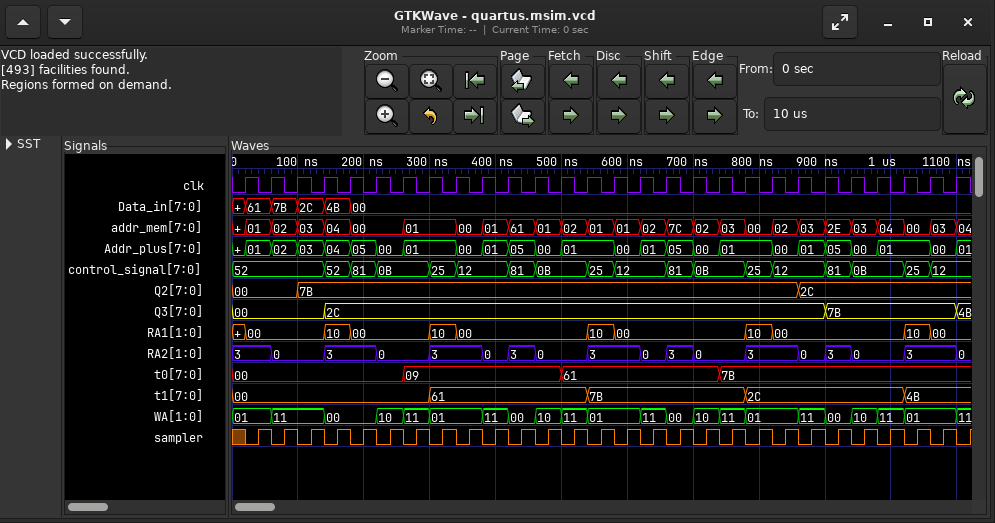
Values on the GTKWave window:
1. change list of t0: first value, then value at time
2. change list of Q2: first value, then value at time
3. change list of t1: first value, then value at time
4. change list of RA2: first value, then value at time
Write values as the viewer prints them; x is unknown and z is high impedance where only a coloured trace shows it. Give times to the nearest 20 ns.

00, 09 at 260 ns, 61 at 500 ns, 7B at 740 ns
00, 7B at 100 ns, 2C at 860 ns
00, 61 at 300 ns, 7B at 540 ns, 2C at 780 ns, 4B at 1020 ns
3, 0 at 60 ns, 3 at 140 ns, 0 at 220 ns, 3 at 300 ns, 0 at 380 ns, 3 at 420 ns, 0 at 460 ns, 3 at 540 ns, 0 at 620 ns, 3 at 660 ns, 0 at 700 ns, 3 at 780 ns, 0 at 860 ns, 3 at 900 ns, 0 at 940 ns, 3 at 1020 ns, 0 at 1100 ns
